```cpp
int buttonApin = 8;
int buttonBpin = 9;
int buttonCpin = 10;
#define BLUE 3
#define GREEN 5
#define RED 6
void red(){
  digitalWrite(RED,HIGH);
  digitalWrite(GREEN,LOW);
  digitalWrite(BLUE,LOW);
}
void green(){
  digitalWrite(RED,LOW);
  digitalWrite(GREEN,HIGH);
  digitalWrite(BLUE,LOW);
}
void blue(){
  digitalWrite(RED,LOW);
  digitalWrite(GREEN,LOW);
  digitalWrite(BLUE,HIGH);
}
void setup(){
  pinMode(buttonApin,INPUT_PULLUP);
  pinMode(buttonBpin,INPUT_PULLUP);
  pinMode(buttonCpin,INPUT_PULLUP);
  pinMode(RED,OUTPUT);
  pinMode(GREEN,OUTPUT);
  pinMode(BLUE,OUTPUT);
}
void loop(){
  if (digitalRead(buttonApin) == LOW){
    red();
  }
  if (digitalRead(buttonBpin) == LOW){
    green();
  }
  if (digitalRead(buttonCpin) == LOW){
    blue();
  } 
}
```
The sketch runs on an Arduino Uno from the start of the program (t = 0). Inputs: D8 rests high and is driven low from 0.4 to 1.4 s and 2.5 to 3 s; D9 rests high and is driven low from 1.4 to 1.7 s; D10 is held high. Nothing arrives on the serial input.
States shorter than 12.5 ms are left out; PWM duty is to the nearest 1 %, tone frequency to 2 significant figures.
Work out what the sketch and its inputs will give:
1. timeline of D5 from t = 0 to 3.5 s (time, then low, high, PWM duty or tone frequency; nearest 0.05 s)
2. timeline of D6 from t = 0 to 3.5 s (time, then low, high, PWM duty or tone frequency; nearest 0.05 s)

0 s low; 1.4 s high; 2.5 s low
0 s low; 0.4 s high; 1.4 s low; 2.5 s high
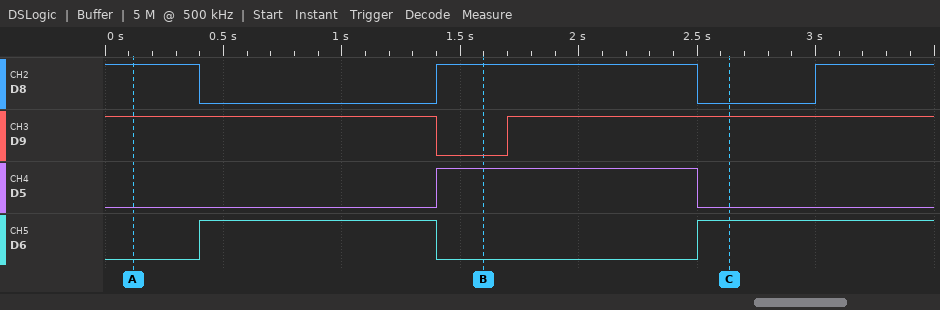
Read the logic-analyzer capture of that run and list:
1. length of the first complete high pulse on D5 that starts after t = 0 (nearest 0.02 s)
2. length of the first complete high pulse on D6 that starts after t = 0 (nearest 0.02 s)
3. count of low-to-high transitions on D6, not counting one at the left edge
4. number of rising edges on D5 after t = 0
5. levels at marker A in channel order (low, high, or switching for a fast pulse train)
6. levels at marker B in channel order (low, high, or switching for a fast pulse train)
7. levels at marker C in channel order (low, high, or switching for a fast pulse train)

1.10 s
1.00 s
2
1
D8 high, D9 high, D5 low, D6 low
D8 high, D9 low, D5 high, D6 low
D8 low, D9 high, D5 low, D6 high
